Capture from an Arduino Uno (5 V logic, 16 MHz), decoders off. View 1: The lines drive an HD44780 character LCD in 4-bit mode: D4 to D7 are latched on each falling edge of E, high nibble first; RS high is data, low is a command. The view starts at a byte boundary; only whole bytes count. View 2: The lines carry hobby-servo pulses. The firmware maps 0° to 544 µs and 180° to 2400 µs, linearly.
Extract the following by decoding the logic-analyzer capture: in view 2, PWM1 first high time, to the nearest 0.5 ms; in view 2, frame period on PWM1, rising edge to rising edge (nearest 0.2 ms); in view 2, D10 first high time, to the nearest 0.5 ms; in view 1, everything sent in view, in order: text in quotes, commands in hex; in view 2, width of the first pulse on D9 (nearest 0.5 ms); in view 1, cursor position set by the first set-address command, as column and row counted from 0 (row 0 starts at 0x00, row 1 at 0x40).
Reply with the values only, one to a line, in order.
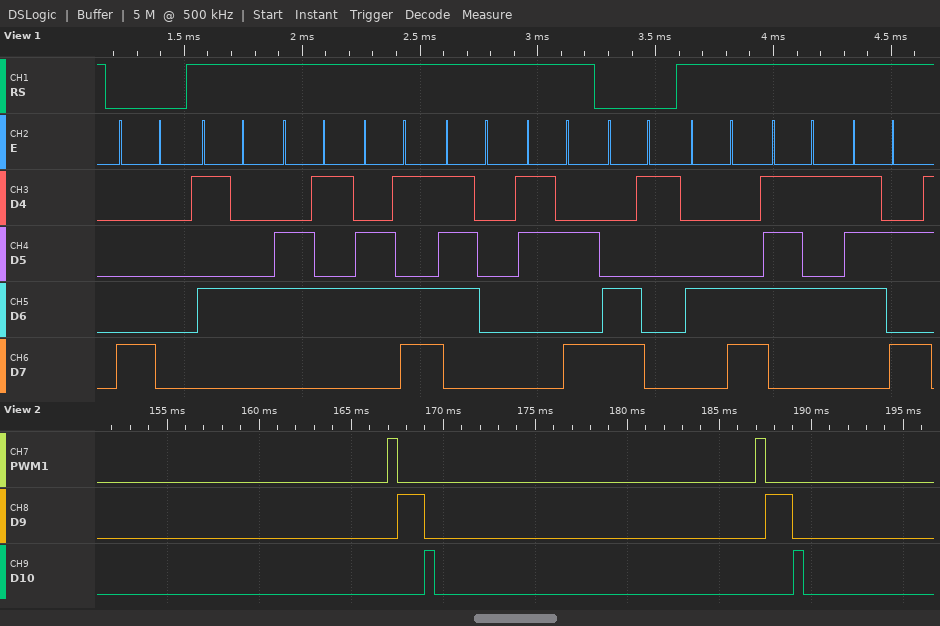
0.5 ms
20.0 ms
0.5 ms
0x80 "Temp:" 0xC1 "Luz"
1.5 ms
column 0, row 0
